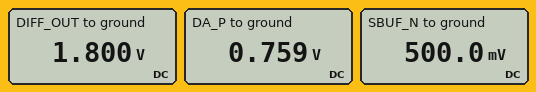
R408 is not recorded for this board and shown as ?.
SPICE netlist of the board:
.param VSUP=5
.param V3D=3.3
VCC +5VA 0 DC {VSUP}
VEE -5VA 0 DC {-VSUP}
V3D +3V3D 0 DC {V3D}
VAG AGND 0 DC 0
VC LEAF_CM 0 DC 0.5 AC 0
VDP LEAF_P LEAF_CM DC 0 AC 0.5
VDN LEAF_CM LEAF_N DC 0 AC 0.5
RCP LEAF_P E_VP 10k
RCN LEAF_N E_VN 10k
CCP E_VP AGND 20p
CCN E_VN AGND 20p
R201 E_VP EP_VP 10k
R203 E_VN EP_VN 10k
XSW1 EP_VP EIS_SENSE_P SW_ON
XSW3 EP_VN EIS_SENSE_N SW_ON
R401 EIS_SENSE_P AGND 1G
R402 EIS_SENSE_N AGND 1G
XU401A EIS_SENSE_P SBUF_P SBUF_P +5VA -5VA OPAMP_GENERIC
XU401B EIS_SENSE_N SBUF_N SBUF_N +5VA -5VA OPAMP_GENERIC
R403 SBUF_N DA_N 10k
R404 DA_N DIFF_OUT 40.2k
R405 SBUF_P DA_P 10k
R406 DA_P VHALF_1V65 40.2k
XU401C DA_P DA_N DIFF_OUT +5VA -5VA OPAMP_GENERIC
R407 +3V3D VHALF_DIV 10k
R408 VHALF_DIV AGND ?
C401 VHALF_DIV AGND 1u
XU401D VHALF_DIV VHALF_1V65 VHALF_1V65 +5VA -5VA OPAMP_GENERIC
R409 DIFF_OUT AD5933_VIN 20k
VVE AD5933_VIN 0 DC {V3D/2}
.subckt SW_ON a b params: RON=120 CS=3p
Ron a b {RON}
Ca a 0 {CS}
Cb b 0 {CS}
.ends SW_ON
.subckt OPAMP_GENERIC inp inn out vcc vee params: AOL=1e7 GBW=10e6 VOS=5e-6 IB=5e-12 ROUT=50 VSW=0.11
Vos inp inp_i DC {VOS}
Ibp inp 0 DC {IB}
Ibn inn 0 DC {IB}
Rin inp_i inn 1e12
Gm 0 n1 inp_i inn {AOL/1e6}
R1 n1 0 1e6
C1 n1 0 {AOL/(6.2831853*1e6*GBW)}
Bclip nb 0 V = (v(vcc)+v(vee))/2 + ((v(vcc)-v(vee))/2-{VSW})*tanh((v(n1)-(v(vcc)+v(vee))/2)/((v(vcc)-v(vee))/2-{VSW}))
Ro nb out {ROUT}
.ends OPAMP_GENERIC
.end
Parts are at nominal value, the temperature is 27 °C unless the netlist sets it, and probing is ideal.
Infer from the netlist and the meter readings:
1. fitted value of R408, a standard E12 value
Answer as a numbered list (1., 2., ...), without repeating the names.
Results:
1. 12 kΩ
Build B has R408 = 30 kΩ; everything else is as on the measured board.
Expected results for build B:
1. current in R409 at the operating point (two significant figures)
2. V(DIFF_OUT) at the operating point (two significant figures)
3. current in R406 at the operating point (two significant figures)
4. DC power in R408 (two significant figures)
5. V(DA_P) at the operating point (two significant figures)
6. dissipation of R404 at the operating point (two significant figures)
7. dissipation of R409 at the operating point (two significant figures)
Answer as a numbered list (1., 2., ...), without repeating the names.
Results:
1. 41 µA
2. 2.5 V
3. 39 µA
4. 200 µW
5. 890 mV
6. 62 µW
7. 34 µW
